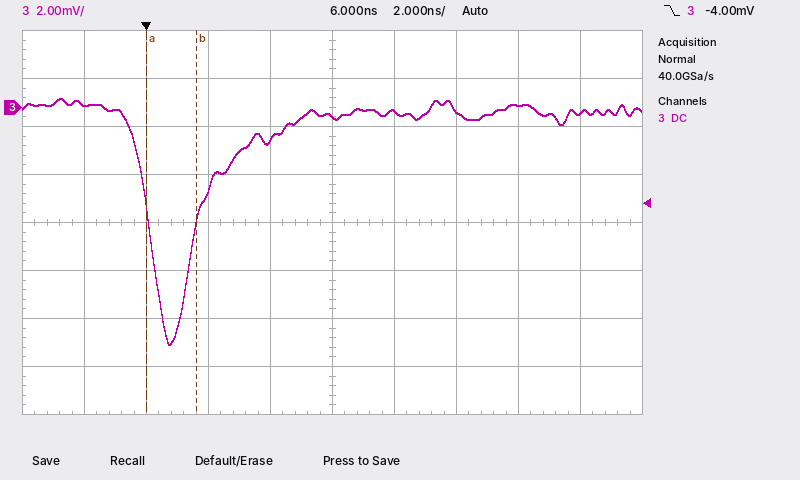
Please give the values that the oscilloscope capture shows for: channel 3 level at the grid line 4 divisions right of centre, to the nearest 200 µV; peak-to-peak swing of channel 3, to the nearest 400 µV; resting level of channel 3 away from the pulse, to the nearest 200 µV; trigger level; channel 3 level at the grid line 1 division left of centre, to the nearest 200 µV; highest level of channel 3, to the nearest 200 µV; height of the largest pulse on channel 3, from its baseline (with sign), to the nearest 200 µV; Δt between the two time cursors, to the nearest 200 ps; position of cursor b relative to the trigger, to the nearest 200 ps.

-200 µV
10.4 mV
-200 µV
-4.00 mV
-1.4 mV
400 µV
-9.6 mV
1.6 ns
+1.6 ns
